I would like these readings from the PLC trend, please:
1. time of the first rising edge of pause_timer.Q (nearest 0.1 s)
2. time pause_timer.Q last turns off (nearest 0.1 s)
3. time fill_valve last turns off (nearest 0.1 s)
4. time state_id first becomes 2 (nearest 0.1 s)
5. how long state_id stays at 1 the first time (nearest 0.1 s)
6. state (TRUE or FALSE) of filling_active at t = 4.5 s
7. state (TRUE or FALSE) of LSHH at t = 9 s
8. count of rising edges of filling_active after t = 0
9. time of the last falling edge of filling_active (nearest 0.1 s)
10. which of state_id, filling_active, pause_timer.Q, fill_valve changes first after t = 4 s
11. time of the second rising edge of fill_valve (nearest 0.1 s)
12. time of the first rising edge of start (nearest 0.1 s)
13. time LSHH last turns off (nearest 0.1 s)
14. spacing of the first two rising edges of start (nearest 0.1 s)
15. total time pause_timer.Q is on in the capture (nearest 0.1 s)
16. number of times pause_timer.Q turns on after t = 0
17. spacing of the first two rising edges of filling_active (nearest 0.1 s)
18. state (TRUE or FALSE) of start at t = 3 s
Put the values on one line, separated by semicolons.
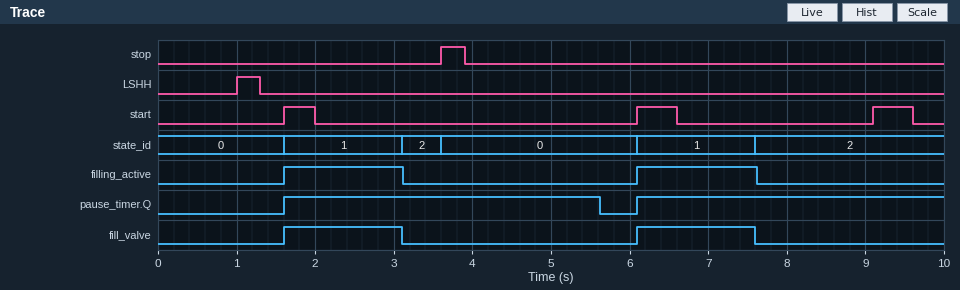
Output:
1.6 s; 5.6 s; 7.6 s; 3.1 s; 1.5 s; FALSE; FALSE; 2; 7.6 s; pause_timer.Q; 6.1 s; 1.6 s; 1.3 s; 4.5 s; 7.9 s; 2; 4.5 s; FALSE
